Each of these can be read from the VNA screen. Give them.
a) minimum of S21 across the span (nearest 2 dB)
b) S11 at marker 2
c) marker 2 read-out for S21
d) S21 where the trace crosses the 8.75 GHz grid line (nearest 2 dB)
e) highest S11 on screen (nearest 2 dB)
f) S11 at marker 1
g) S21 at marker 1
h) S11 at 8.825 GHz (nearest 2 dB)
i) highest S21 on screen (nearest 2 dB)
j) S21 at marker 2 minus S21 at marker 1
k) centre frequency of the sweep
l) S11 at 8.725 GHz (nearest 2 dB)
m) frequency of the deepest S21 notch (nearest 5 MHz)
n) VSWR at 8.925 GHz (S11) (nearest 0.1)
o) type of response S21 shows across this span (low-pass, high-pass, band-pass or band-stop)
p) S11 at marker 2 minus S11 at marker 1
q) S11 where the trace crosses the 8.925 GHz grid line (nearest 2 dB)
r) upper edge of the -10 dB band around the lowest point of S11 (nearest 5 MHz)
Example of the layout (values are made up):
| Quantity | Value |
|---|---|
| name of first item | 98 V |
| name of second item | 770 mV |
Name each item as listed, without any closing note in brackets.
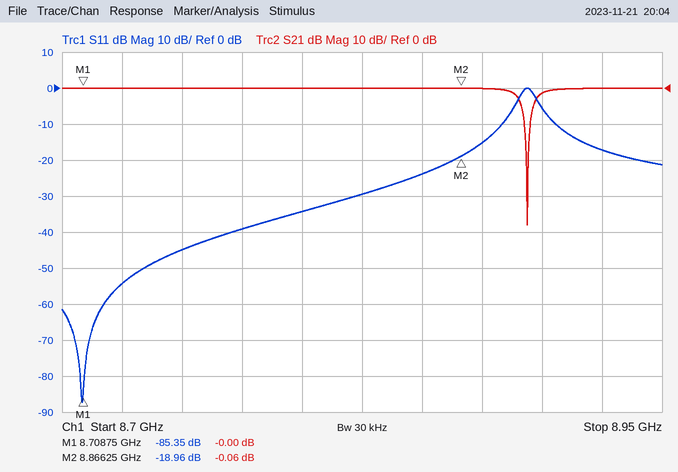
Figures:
| Quantity | Value |
|---|---|
| minimum of S21 across the span | -38 dB |
| S11 at marker 2 | -18.96 dB |
| marker 2 read-out for S21 | -0.06 dB |
| S21 where the trace crosses the 8.75 GHz grid line | 0 dB |
| highest S11 on screen | 0 dB |
| S11 at marker 1 | -85.35 dB |
| S21 at marker 1 | -0.00 dB |
| S11 at 8.825 GHz | -30 dB |
| highest S21 on screen | 0 dB |
| S21 at marker 2 minus S21 at marker 1 | -0.06 dB |
| centre frequency of the sweep | 8.825 GHz |
| S11 at 8.725 GHz | -54 dB |
| frequency of the deepest S21 notch | 8.895 GHz |
| VSWR at 8.925 GHz (S11) | 1.3 |
| type of response S21 shows across this span | band-stop |
| S11 at marker 2 minus S11 at marker 1 | 66.39 dB |
| S11 where the trace crosses the 8.925 GHz grid line | -18 dB |
| upper edge of the -10 dB band around the lowest point of S11 | 8.885 GHz |
